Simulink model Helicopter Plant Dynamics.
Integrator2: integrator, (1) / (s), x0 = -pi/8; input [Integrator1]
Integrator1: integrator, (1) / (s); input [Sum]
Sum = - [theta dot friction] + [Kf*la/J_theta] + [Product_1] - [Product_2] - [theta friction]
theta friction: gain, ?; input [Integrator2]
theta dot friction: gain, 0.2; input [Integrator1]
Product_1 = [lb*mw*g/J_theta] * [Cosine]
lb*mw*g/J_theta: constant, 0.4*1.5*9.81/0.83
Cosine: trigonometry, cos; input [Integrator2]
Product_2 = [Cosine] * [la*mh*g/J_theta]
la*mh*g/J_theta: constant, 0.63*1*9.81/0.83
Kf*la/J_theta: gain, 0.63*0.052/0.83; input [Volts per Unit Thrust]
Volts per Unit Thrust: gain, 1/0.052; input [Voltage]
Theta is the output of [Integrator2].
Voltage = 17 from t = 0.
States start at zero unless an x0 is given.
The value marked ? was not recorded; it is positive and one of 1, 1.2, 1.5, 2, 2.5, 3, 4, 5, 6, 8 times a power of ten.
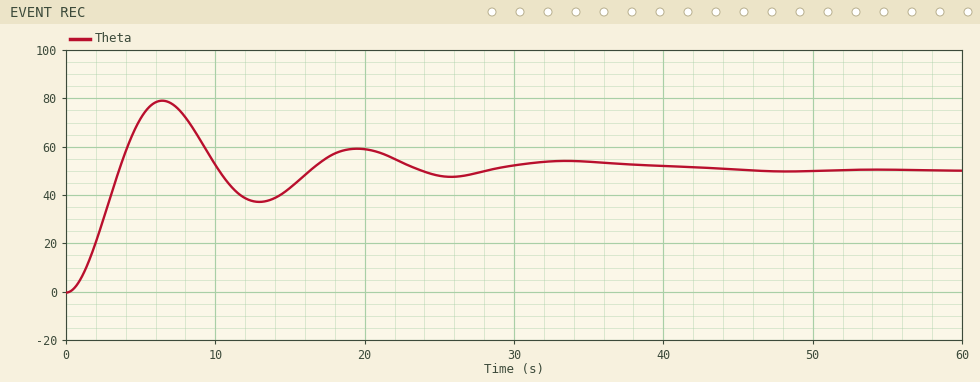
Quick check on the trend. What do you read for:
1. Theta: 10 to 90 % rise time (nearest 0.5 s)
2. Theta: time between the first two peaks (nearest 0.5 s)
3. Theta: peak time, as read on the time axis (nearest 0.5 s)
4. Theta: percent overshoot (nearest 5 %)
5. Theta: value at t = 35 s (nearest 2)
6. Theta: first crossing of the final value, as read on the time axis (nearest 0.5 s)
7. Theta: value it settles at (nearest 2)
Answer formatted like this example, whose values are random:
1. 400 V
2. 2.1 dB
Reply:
1. 2.5 s
2. 13.0 s
3. 6.5 s
4. 55 %
5. 54
6. 3.5 s
7. 50
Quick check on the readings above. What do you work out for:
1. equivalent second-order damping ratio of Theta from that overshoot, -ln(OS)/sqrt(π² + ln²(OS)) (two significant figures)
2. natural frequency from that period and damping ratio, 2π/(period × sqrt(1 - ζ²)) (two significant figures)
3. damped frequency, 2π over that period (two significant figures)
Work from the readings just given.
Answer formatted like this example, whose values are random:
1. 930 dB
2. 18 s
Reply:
1. 0.19
2. 0.49 rad/s
3. 0.48 rad/s
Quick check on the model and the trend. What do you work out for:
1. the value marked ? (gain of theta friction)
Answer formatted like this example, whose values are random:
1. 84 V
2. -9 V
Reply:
1. 0.25
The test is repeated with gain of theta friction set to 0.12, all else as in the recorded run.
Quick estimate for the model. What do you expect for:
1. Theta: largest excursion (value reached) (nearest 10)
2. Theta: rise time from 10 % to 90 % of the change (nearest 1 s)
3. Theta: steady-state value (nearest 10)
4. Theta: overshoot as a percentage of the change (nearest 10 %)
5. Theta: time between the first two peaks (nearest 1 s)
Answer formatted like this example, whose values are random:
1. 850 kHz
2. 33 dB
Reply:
1. 150
2. 4 s
3. 110
4. 40 %
5. 18 s
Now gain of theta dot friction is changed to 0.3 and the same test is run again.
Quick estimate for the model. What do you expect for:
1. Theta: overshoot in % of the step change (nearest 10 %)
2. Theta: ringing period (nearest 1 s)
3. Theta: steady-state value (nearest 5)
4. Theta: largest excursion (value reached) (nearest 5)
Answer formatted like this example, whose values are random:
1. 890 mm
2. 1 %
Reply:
1. 40 %
2. 14 s
3. 50
4. 70
